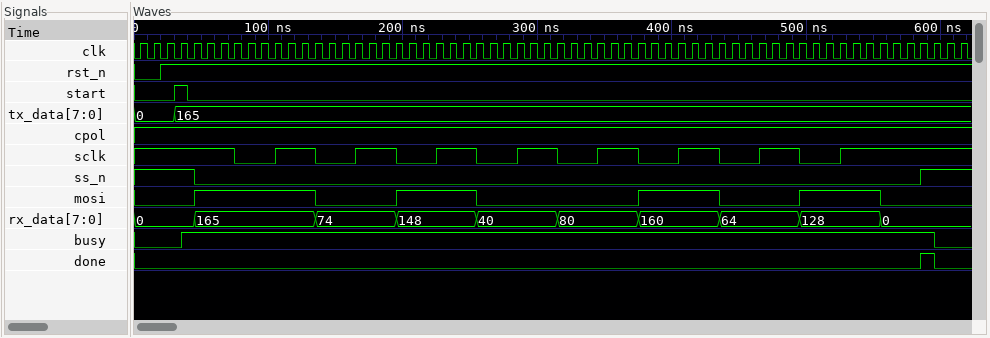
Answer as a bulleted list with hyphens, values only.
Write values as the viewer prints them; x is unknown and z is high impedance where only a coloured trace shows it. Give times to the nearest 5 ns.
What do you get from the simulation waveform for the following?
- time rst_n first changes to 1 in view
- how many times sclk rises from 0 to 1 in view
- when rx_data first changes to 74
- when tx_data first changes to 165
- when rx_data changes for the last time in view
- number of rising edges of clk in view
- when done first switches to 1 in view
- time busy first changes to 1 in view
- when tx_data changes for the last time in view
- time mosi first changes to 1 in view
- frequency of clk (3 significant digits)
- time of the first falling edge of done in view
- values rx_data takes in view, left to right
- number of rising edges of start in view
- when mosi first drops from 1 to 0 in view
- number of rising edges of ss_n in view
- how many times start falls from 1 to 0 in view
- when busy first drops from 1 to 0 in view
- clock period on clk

- 20 ns
- 8
- 135 ns
- 30 ns
- 555 ns
- 62
- 585 ns
- 35 ns
- 30 ns
- 45 ns
- 100 MHz
- 595 ns
- 0, 165, 74, 148, 40, 80, 160, 64, 128, 0
- 1
- 135 ns
- 1
- 1
- 595 ns
- 10 ns
